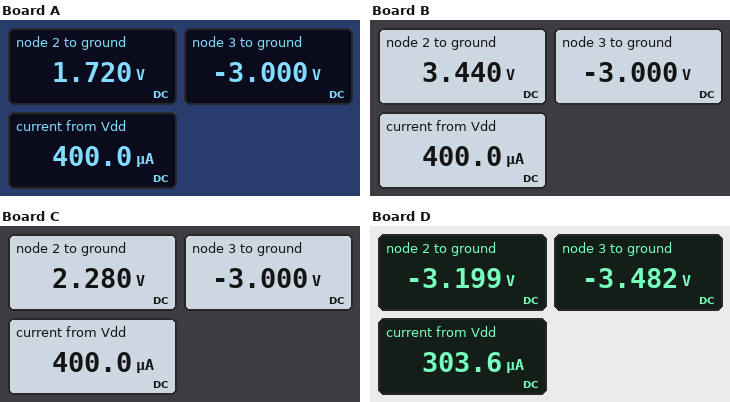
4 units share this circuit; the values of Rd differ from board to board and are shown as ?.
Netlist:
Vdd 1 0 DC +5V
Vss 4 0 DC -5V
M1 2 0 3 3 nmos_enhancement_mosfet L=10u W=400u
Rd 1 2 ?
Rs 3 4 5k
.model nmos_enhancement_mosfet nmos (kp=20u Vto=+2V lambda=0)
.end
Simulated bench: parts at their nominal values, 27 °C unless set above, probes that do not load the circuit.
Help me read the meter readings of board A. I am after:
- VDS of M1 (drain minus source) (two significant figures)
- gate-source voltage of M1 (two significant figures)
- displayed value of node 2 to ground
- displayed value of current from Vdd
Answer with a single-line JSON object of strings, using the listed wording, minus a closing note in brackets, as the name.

{"VDS of M1 (drain minus source)": "4.7 V", "gate-source voltage of M1": "3.0 V", "displayed value of node 2 to ground": "1.720 V", "displayed value of current from Vdd": "400.0 µA"}
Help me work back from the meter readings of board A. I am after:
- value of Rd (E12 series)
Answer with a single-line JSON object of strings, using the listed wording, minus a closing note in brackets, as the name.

{"value of Rd": "8.2 kΩ"}
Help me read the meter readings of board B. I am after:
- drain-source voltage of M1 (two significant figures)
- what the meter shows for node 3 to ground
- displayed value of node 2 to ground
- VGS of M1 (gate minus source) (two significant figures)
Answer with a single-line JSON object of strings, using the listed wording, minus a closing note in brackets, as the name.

{"drain-source voltage of M1": "6.4 V", "what the meter shows for node 3 to ground": "-3.000 V", "displayed value of node 2 to ground": "3.440 V", "VGS of M1 (gate minus source)": "3.0 V"}
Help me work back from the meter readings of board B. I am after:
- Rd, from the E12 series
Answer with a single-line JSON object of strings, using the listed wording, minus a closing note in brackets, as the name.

{"Rd, from the E12 series": "3.9 kΩ"}
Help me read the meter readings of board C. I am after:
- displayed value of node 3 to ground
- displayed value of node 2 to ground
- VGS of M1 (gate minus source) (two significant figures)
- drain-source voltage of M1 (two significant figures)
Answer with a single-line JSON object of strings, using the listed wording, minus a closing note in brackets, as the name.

{"displayed value of node 3 to ground": "-3.000 V", "displayed value of node 2 to ground": "2.280 V", "VGS of M1 (gate minus source)": "3.0 V", "drain-source voltage of M1": "5.3 V"}
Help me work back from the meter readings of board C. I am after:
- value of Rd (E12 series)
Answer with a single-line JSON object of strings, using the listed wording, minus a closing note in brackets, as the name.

{"value of Rd": "6.8 kΩ"}
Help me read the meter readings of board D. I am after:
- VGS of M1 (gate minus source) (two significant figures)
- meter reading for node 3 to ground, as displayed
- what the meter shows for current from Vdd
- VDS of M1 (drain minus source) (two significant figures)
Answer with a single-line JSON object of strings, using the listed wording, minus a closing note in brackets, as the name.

{"VGS of M1 (gate minus source)": "3.5 V", "meter reading for node 3 to ground, as displayed": "-3.482 V", "what the meter shows for current from Vdd": "303.6 µA", "VDS of M1 (drain minus source)": "280 mV"}
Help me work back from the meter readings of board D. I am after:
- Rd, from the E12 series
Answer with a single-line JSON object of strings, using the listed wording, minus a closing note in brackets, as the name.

{"Rd, from the E12 series": "27 kΩ"}
